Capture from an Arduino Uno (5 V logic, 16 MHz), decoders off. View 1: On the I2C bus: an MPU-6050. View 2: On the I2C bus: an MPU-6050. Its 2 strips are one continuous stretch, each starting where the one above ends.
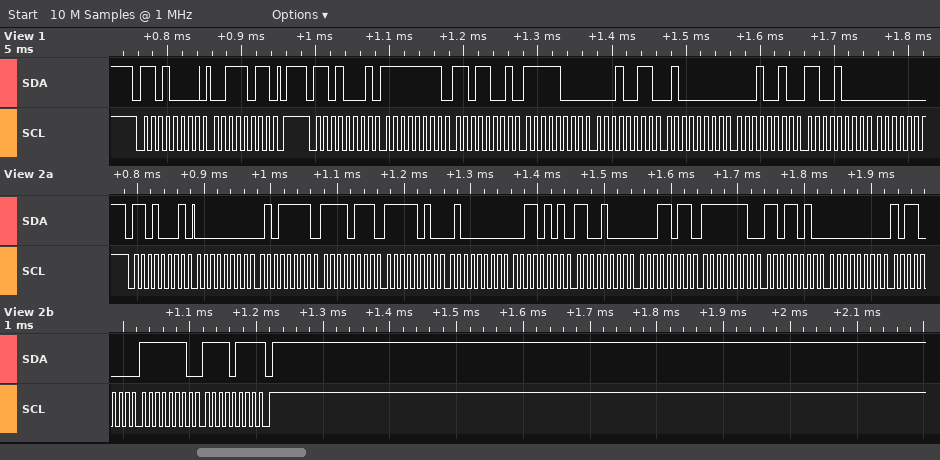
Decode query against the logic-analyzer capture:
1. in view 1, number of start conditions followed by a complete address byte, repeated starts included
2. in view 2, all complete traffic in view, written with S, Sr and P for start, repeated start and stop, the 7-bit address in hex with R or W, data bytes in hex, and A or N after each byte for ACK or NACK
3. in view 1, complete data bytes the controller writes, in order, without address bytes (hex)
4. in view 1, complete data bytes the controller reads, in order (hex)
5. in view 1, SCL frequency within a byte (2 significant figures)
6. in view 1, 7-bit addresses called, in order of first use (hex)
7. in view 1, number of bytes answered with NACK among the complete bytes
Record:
2
S 68R A 00 A 5F A F7 A FA A 40 A 35 A C8 A 1B A FE A DA A 00 A B0 A FE A F7 N P
3B
FF D9 F8 13 40 12 C8
100 kHz
0x68
0
